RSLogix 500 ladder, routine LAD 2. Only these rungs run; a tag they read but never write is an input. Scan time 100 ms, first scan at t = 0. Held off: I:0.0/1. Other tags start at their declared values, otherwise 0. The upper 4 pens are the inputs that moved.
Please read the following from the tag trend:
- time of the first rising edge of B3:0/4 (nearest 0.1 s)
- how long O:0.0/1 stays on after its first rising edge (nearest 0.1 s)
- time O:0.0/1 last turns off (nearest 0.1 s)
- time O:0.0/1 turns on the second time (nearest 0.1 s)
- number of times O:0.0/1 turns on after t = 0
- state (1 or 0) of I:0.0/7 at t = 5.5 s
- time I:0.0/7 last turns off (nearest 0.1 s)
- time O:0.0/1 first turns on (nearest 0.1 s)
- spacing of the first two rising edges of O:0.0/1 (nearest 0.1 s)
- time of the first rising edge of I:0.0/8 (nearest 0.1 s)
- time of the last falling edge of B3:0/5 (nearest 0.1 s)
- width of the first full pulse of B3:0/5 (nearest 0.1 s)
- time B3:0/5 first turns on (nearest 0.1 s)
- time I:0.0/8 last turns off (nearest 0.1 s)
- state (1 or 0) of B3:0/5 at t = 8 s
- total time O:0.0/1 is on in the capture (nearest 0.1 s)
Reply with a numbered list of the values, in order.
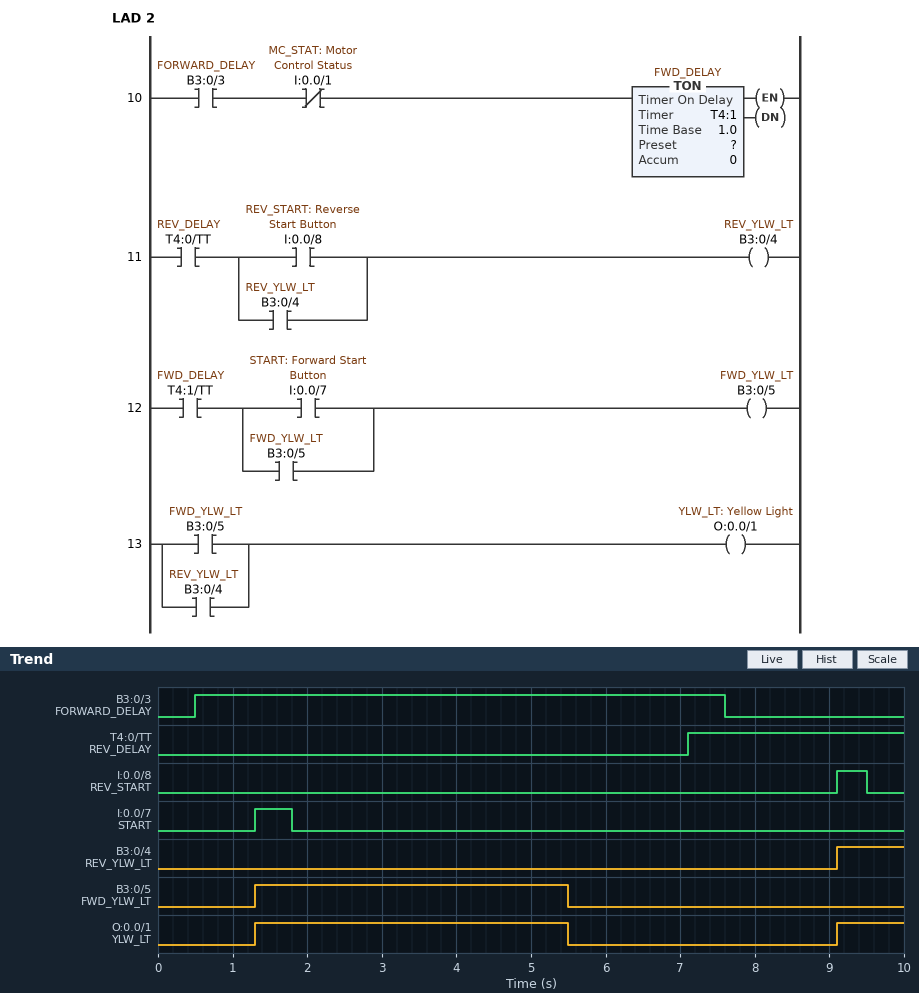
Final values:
1. 9.1 s
2. 4.2 s
3. 5.5 s
4. 9.1 s
5. 2
6. 0
7. 1.8 s
8. 1.3 s
9. 7.8 s
10. 9.1 s
11. 5.5 s
12. 4.2 s
13. 1.3 s
14. 9.5 s
15. 0
16. 5.1 s
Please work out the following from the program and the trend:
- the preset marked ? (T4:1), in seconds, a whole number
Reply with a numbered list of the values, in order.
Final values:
1. 5 s
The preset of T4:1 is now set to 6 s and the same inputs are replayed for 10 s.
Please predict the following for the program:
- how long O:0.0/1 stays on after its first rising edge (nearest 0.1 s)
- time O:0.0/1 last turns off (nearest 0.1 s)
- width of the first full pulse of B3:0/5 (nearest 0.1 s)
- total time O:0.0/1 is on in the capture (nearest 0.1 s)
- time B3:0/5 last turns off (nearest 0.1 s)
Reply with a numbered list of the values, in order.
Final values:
1. 5.2 s
2. 6.5 s
3. 5.2 s
4. 6.1 s
5. 6.5 s
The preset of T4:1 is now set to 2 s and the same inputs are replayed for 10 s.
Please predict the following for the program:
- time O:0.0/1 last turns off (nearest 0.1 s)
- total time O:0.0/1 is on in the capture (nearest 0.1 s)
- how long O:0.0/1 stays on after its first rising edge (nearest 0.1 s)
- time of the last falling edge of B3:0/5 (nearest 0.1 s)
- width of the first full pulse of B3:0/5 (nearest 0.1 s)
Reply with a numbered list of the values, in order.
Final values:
1. 2.5 s
2. 2.1 s
3. 1.2 s
4. 2.5 s
5. 1.2 s
